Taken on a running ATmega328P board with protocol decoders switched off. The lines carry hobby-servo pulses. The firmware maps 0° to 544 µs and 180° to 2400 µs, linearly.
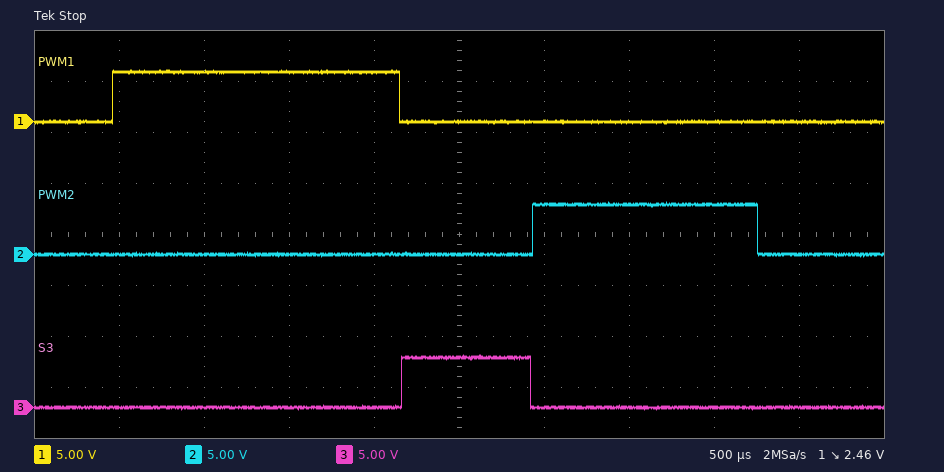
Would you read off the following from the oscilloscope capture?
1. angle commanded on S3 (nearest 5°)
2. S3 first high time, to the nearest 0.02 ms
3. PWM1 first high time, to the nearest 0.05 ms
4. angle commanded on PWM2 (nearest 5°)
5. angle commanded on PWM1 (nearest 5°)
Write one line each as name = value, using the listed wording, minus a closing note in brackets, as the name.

angle commanded on S3 = 20°
S3 first high time, to the nearest 0.02 ms = 0.76 ms
PWM1 first high time, to the nearest 0.05 ms = 1.70 ms
angle commanded on PWM2 = 75°
angle commanded on PWM1 = 110°
